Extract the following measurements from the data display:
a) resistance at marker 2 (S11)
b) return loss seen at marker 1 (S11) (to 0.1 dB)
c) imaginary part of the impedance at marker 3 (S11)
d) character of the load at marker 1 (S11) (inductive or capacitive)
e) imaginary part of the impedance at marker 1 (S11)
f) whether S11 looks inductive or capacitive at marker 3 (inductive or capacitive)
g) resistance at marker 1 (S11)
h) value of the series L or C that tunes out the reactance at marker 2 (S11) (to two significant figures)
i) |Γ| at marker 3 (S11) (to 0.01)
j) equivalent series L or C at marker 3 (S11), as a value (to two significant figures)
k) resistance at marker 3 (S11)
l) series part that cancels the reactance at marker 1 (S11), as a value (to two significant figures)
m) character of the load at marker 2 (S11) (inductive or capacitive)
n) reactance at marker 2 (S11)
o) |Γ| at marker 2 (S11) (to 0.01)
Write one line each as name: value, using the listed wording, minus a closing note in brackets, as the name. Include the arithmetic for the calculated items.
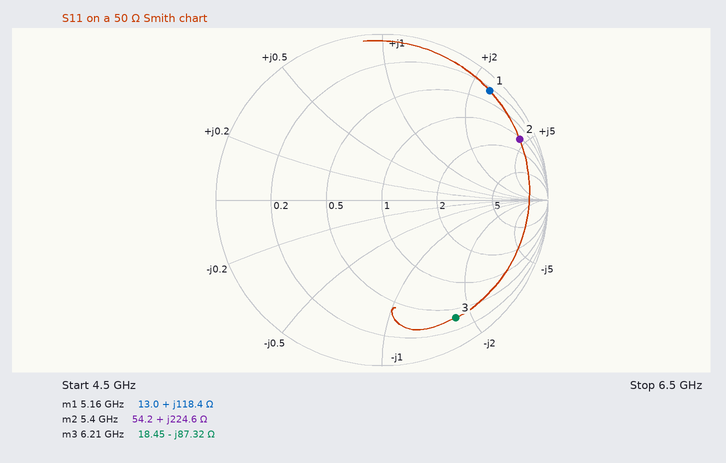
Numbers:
resistance at marker 2: 54.2 Ω
return loss seen at marker 1 (S11): 0.7 dB
imaginary part of the impedance at marker 3: -87.32 Ω
character of the load at marker 1 (S11): inductive
imaginary part of the impedance at marker 1: +118.4 Ω
whether S11 looks inductive or capacitive at marker 3: capacitive
resistance at marker 1: 13.0 Ω
value of the series L or C that tunes out the reactance at marker 2 (S11): C = 1/(2π × 5.4 GHz × 224.6 Ω) ≈ 131 fF, so 130 fF to two significant figures
|Γ| at marker 3 (S11): 0.84
equivalent series L or C at marker 3 (S11), as a value: C = 1/(2π × 6.21 GHz × 87.32 Ω) ≈ 294 fF, so 290 fF to two significant figures
resistance at marker 3: 18.45 Ω
series part that cancels the reactance at marker 1 (S11), as a value: C = 1/(2π × 5.16 GHz × 118.4 Ω) ≈ 261 fF, so 260 fF to two significant figures
character of the load at marker 2 (S11): inductive
reactance at marker 2: +224.6 Ω
|Γ| at marker 2 (S11): 0.91
